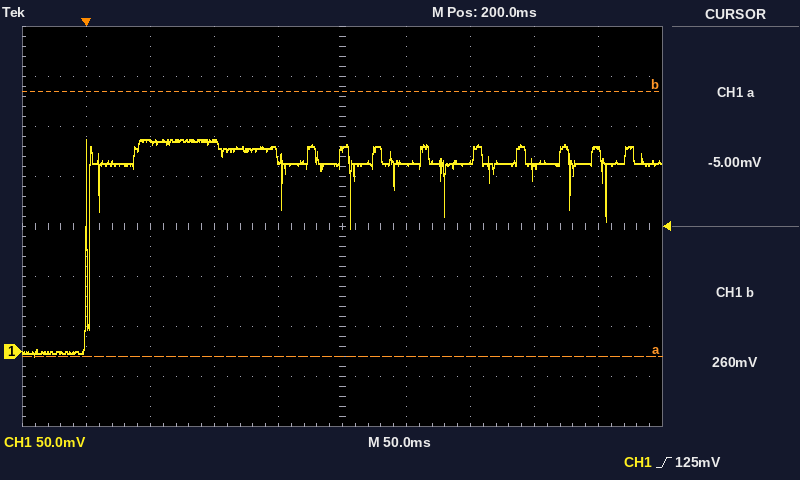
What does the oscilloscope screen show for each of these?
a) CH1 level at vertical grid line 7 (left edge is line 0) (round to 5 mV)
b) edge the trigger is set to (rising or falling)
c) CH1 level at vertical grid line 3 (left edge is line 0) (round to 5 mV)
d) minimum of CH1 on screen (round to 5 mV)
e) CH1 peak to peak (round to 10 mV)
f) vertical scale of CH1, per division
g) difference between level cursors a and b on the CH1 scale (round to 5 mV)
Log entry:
190 mV
rising
210 mV
-5 mV
220 mV
50 mV
265 mV
